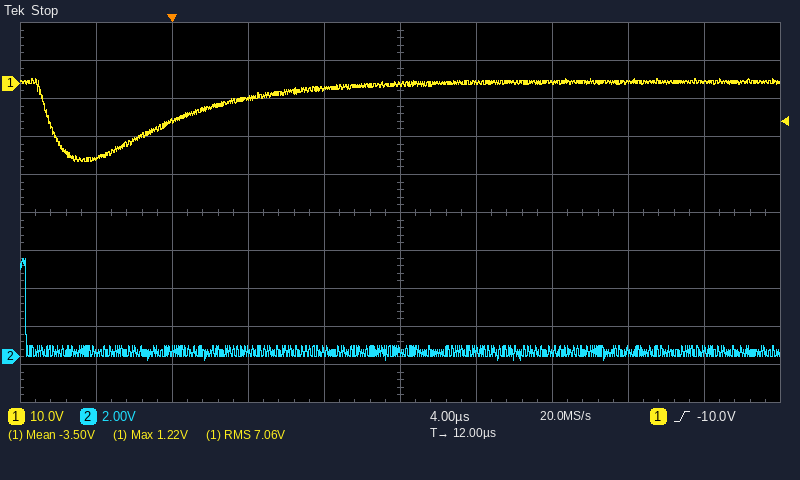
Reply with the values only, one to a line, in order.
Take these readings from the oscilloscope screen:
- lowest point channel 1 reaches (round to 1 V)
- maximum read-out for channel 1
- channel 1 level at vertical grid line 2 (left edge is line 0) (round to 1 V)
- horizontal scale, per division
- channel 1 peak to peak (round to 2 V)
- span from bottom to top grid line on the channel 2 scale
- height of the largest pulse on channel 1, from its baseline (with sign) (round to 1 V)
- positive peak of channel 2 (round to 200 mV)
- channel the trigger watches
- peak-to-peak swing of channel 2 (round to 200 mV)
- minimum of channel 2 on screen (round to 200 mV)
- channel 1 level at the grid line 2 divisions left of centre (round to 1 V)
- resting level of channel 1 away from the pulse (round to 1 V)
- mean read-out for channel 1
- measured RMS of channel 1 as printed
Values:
-21 V
1.22 V
-10 V
4 µs
22 V
20 V
-21 V
5.2 V
channel 1
5.4 V
-200 mV
-4 V
0 V
-3.50 V
7.06 V
